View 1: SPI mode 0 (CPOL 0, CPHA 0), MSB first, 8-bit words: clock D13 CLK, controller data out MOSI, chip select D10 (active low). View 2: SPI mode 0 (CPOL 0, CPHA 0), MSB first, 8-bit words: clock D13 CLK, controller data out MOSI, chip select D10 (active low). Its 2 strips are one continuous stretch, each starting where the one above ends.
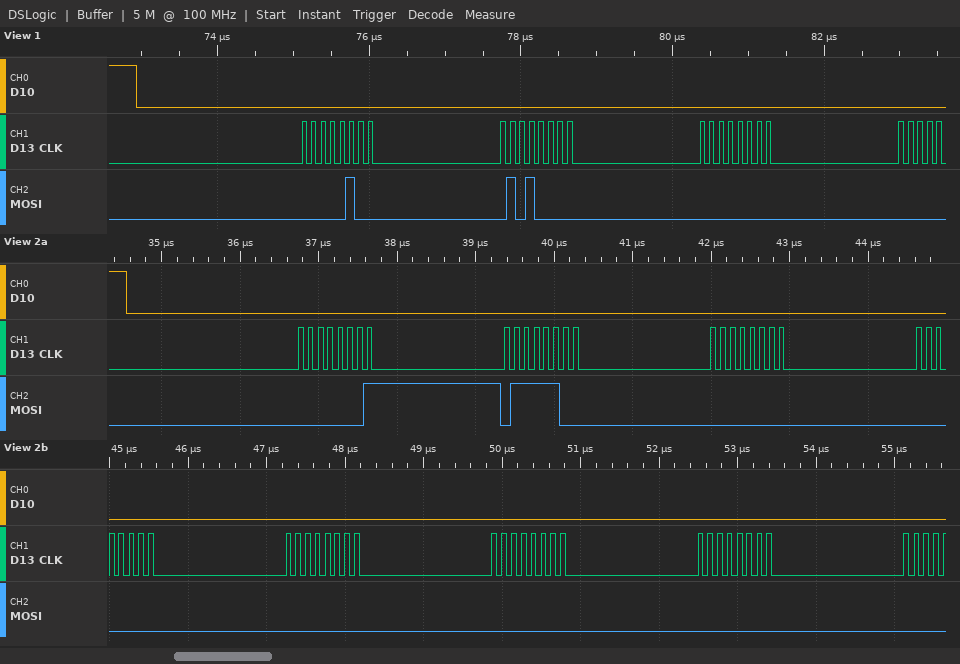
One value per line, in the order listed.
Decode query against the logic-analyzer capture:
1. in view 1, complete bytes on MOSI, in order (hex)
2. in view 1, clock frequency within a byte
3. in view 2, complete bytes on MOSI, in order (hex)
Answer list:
04 50 00
8 MHz
0x01 0x7C 0x00 0x00 0x00 0x00 0x00
